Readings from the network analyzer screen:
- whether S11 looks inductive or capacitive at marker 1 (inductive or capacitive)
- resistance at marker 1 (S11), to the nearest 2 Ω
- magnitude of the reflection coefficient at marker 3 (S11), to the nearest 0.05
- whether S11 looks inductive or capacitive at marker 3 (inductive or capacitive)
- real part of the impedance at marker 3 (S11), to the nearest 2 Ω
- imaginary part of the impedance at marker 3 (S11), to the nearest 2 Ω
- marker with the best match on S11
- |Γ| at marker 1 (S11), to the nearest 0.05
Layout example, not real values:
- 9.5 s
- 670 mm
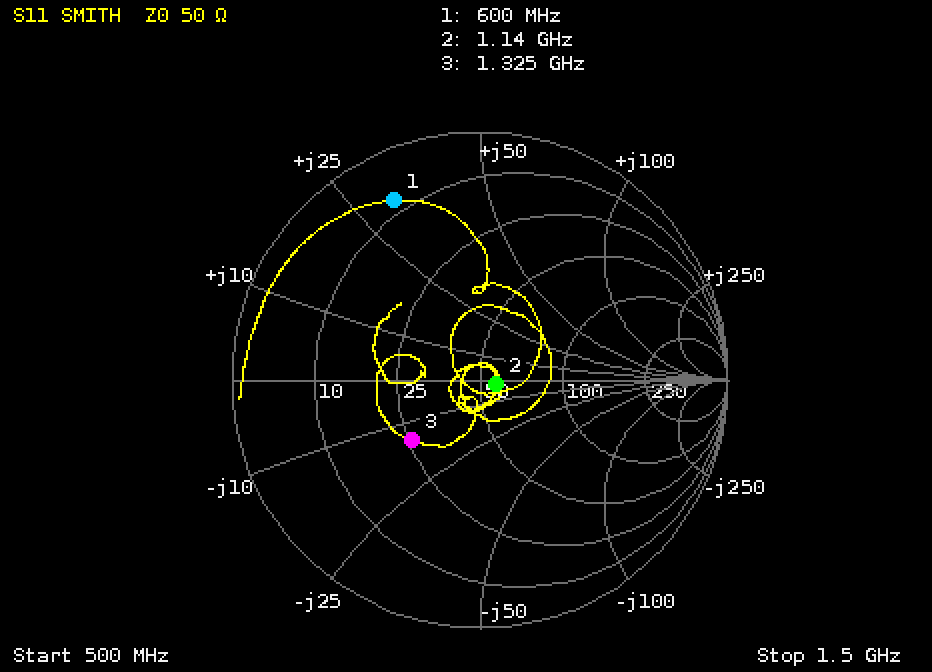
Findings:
- inductive
- 8 Ω
- 0.35
- capacitive
- 26 Ω
- -14 Ω
- marker 2
- 0.80
